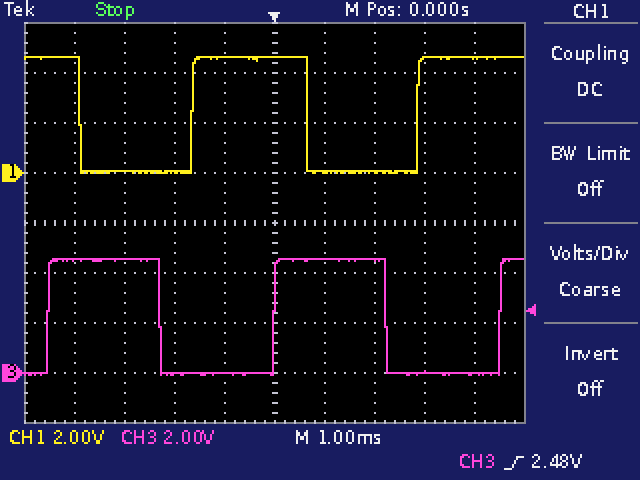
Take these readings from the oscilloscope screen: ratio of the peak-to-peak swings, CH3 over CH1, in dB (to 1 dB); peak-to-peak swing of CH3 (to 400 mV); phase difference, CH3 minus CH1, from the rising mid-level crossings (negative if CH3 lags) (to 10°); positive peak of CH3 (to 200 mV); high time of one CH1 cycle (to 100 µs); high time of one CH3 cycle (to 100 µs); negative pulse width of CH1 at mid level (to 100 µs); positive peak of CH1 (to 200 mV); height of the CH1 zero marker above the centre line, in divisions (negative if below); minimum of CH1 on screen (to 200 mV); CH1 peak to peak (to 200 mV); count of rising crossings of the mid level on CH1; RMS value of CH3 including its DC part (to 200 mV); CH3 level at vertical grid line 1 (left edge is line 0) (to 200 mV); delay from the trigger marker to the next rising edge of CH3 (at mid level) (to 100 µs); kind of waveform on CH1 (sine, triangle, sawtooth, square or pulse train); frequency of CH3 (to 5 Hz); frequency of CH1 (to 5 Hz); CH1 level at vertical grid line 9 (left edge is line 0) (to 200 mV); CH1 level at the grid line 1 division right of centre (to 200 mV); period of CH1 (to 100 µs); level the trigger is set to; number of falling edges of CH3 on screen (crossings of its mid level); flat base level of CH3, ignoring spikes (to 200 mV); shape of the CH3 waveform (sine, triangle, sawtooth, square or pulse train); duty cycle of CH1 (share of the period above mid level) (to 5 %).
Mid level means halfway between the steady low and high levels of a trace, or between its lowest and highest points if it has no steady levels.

0 dB
4.8 V
-130°
4.6 V
2.3 ms
2.2 ms
2.2 ms
4.6 V
+1.0 div
0.0 V
4.6 V
2
3.2 V
4.6 V
4.5 ms
square
220 Hz
220 Hz
4.6 V
0.0 V
4.5 ms
2.48 V
2
0.0 V
square
50 %
